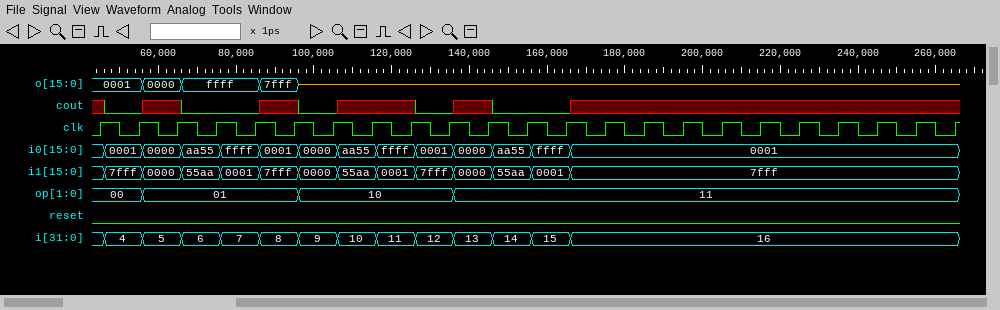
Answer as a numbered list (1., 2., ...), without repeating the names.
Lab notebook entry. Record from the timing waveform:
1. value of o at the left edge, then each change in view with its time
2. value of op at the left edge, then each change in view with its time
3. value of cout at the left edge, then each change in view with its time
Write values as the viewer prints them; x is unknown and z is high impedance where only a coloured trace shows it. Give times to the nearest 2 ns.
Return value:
1. 0001, 0000 at 56 ns, ffff at 66 ns, 7fff at 86 ns, z at 96 ns
2. 00, 01 at 56 ns, 10 at 96 ns, 11 at 136 ns
3. x, 0 at 46 ns, x at 56 ns, 0 at 66 ns, x at 86 ns, 0 at 96 ns, x at 106 ns, 0 at 126 ns, x at 136 ns, 0 at 146 ns, x at 166 ns
